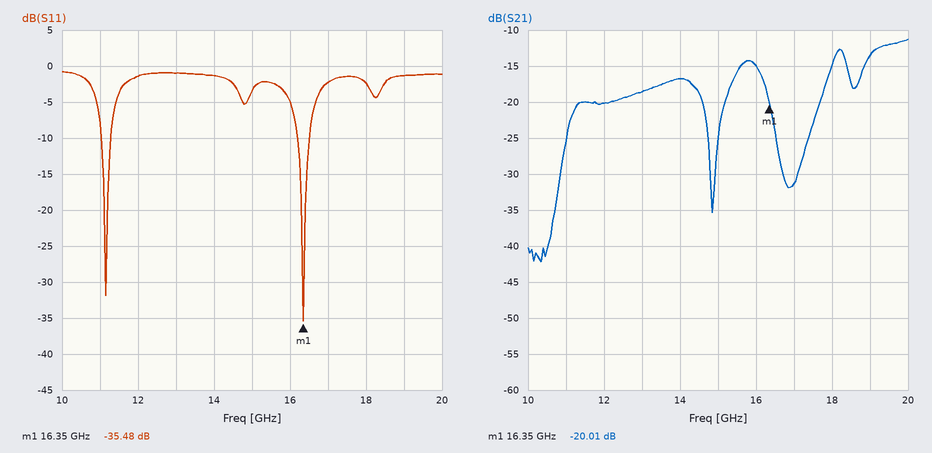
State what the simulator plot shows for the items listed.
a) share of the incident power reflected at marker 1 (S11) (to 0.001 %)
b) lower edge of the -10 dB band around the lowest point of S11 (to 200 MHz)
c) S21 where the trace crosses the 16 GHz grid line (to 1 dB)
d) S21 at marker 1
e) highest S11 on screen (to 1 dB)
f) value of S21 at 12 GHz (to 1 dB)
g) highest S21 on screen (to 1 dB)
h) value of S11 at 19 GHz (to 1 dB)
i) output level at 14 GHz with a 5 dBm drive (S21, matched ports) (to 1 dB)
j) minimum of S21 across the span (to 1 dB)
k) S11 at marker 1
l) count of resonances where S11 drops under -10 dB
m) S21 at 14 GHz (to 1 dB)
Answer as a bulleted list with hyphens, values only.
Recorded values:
- 0.028 %
- 16.2 GHz
- -15 dB
- -20.01 dB
- -1 dB
- -20 dB
- -11 dB
- -1 dB
- -12 dBm
- -42 dB
- -35.48 dB
- 2
- -17 dB
